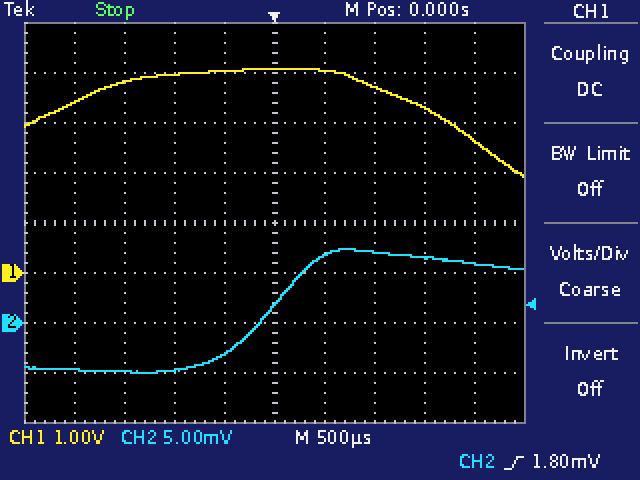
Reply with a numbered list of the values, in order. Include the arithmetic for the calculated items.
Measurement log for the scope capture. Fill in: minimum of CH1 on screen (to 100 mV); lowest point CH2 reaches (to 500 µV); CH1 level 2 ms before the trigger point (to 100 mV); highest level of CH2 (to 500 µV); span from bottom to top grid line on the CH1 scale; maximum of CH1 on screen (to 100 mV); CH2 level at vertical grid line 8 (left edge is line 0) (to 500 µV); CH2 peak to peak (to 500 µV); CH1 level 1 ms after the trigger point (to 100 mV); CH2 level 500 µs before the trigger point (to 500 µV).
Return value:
1. 1.9 V
2. -5.0 mV
3. 3.4 V
4. 7.5 mV
5. 8 V
6. 4.1 V
7. 6.5 mV
8. 7.5 mV − (-5.0 mV) = 12.5 mV
9. 3.7 V
10. -3.0 mV
